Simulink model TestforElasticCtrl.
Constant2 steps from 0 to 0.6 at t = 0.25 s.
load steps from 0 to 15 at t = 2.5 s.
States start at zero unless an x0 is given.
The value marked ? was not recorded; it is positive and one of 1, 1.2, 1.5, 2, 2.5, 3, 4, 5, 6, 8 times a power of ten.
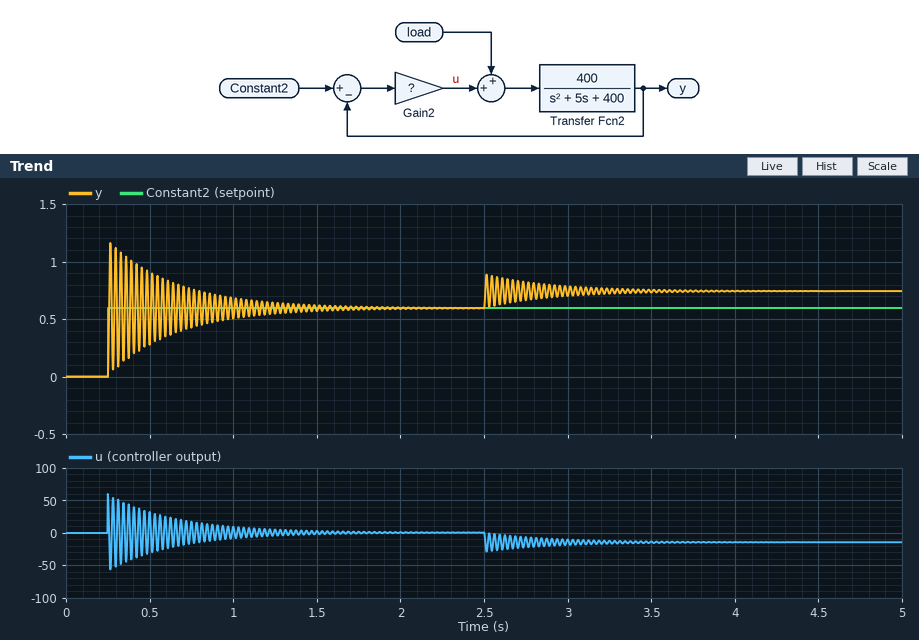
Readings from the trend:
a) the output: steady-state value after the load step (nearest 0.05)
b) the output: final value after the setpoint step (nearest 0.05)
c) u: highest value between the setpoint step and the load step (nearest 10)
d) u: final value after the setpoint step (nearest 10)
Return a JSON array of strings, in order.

["0.75", "0.60", "60", "0"]
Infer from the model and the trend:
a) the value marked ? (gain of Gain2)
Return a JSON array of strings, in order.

["100"]
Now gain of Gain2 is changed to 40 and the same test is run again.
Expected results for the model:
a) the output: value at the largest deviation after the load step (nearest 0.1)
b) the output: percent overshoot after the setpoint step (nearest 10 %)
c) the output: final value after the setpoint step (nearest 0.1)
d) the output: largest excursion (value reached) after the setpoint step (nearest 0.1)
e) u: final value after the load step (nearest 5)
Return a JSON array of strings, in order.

["1.3", "90 %", "0.6", "1.1", "-15"]
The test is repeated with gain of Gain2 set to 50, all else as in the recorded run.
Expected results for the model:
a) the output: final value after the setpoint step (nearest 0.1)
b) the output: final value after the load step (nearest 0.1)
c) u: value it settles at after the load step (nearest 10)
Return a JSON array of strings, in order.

["0.6", "0.9", "-10"]
